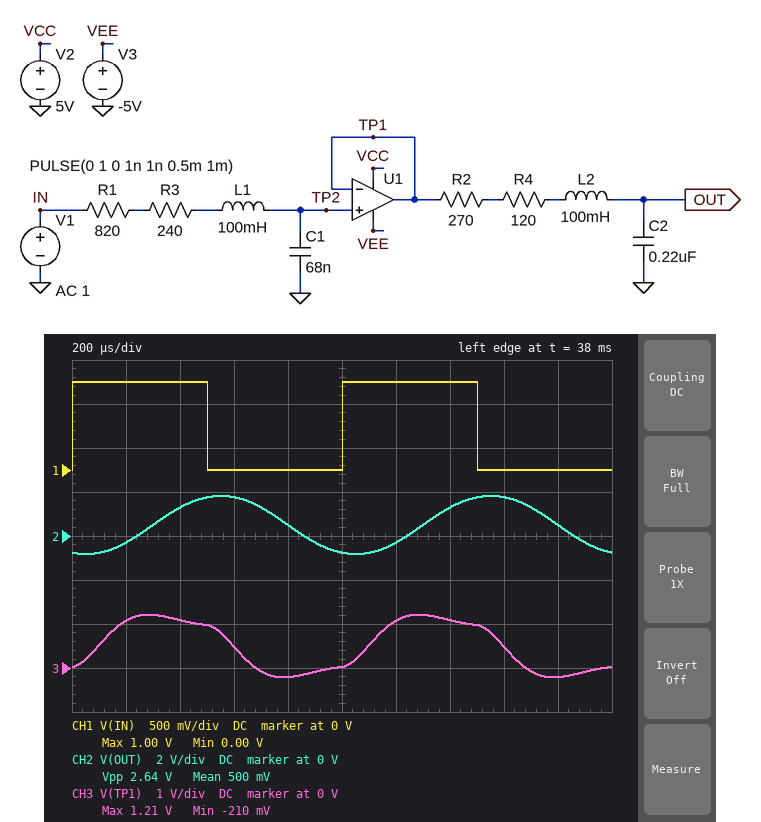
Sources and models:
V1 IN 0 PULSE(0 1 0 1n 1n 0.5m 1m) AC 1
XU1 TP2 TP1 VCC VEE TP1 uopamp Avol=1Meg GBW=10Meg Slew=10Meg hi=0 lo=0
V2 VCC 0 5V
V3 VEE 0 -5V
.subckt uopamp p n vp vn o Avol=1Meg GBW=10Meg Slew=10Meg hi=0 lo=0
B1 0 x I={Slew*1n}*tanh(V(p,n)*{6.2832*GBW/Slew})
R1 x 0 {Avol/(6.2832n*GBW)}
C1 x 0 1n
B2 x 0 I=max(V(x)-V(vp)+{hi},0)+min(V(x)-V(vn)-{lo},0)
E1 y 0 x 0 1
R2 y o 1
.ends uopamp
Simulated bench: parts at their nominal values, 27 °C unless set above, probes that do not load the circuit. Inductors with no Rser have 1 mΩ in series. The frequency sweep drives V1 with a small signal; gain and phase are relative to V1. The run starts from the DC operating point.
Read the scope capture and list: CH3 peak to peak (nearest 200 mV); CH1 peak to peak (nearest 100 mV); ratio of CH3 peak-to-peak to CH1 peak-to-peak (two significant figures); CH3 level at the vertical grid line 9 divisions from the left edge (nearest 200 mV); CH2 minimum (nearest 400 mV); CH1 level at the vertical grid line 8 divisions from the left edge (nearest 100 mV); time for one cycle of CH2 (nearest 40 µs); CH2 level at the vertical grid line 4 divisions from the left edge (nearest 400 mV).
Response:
1.4 V
1.0 V
1.4
-200 mV
-800 mV
0 V
1.00 ms
400 mV
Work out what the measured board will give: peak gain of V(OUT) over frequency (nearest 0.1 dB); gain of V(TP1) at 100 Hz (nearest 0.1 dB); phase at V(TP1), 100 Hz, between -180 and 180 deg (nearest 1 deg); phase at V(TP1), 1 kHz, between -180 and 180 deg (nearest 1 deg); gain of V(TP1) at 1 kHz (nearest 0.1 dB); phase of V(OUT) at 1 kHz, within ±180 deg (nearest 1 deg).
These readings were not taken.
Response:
6.4 dB
0 dB
-3 deg
-32 deg
1.3 dB
-108 deg
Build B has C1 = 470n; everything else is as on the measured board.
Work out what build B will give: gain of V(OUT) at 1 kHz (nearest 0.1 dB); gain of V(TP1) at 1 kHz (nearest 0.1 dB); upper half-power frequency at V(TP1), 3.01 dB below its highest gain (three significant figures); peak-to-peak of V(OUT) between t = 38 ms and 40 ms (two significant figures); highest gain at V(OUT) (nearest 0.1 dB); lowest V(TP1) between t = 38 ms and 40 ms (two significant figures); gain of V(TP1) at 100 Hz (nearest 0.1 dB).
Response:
-5.1 dB
-10.2 dB
389 Hz
710 mV
0 dB
290 mV
-0.3 dB
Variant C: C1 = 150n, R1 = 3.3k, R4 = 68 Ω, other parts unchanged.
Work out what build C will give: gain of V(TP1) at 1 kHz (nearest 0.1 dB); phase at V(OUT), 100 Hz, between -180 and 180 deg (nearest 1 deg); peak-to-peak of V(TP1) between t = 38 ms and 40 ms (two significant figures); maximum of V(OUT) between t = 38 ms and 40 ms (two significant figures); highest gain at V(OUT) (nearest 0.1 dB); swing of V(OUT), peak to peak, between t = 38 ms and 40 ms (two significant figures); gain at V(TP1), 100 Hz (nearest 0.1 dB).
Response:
-10.5 dB
-21 deg
430 mV
890 mV
0 dB
790 mV
-0.4 dB
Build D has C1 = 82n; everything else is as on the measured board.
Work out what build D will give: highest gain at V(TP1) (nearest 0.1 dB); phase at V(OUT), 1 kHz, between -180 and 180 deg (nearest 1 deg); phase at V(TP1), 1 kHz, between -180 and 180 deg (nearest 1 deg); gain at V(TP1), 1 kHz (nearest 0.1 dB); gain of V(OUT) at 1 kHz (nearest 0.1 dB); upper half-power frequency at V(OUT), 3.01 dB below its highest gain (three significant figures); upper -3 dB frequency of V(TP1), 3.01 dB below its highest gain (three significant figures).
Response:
1.5 dB
-115 deg
-39 deg
1.2 dB
6.3 dB
1.28 kHz
2.07 kHz
